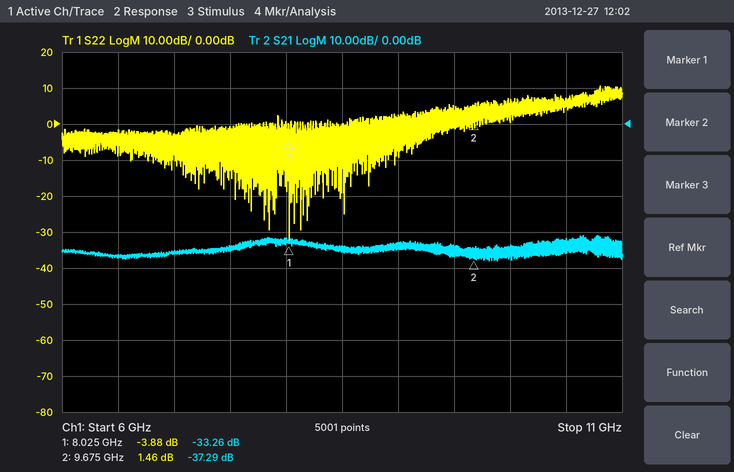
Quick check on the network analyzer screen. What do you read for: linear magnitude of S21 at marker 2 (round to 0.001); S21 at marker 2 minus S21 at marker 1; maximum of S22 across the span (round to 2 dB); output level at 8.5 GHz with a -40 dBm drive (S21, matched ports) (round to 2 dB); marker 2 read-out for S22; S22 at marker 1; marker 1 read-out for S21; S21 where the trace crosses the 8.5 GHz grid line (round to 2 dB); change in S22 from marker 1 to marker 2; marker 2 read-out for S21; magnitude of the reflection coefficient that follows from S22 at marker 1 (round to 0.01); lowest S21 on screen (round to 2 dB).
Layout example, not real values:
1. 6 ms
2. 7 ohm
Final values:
1. 0.014
2. -4.03 dB
3. 10 dB
4. -74 dBm
5. 1.46 dB
6. -3.88 dB
7. -33.26 dB
8. -34 dB
9. 5.34 dB
10. -37.29 dB
11. 0.64
12. -38 dB
